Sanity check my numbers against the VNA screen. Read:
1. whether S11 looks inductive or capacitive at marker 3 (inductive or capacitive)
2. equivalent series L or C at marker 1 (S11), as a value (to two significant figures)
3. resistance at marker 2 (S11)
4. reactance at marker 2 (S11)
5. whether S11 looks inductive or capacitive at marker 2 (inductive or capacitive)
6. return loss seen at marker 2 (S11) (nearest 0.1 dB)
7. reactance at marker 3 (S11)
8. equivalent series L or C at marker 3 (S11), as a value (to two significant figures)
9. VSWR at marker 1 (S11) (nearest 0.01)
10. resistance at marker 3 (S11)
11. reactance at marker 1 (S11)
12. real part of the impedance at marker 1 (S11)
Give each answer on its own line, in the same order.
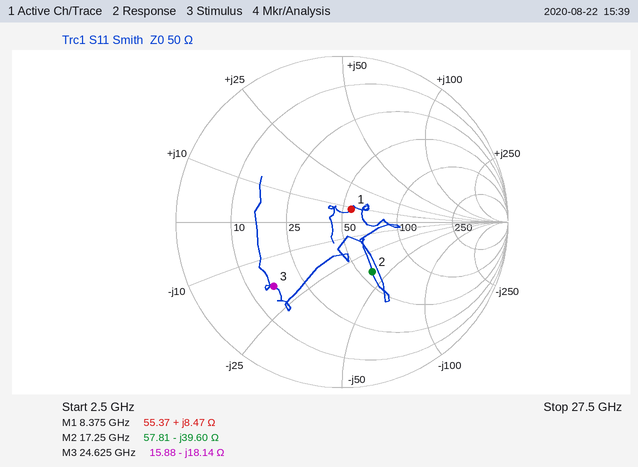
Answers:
capacitive
160 pH
57.81 Ω
-39.60 Ω
capacitive
9.1 dB
-18.14 Ω
360 fF
1.21
15.88 Ω
+8.47 Ω
55.37 Ω
